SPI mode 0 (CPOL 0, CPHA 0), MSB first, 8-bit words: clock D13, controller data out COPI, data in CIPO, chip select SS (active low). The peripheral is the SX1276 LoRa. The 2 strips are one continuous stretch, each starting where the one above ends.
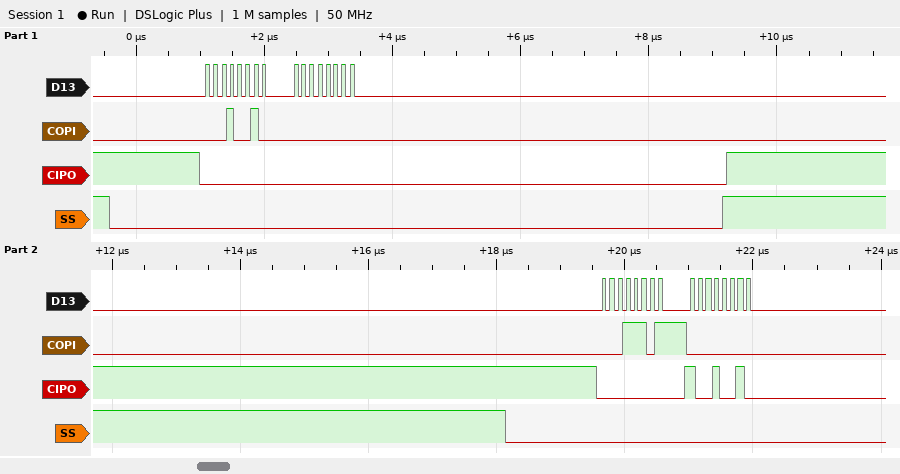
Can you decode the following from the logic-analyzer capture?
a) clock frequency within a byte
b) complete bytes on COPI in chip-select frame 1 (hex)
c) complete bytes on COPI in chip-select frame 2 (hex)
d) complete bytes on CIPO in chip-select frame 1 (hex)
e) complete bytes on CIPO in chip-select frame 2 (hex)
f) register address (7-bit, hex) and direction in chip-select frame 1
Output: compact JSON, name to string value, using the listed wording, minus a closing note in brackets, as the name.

{"clock frequency within a byte": "8 MHz", "complete bytes on COPI in chip-select frame 1": "12 00", "complete bytes on COPI in chip-select frame 2": "1D 00", "complete bytes on CIPO in chip-select frame 1": "00 00", "complete bytes on CIPO in chip-select frame 2": "00 92", "register address (7-bit, hex) and direction in chip-select frame 1": "0x12 read"}
